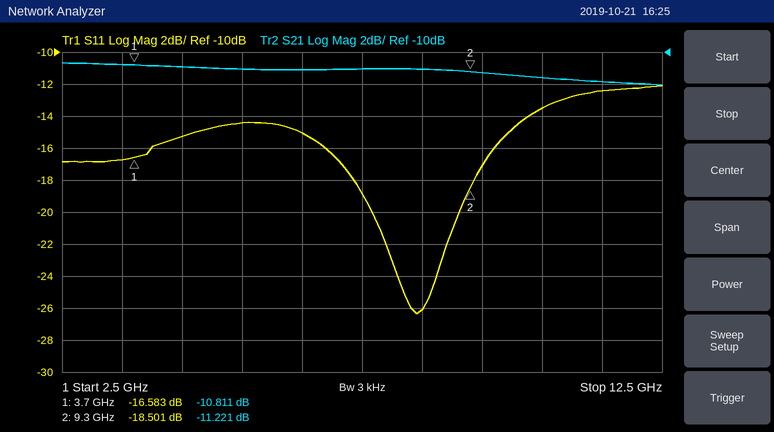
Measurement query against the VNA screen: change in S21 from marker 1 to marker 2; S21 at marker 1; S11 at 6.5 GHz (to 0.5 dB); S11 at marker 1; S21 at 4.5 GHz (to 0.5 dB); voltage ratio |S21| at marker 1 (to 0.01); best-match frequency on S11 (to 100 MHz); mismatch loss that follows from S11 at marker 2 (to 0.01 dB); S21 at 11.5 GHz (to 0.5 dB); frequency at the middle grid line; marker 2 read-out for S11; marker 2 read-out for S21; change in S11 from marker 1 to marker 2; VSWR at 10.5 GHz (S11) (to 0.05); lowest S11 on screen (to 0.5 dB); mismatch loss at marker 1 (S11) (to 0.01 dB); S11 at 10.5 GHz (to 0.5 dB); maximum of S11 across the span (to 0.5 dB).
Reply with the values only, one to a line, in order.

-0.410 dB
-10.811 dB
-15.0 dB
-16.583 dB
-11.0 dB
0.29
8.4 GHz
0.06 dB
-12.0 dB
7.5 GHz
-18.501 dB
-11.221 dB
-1.918 dB
1.55
-26.5 dB
0.10 dB
-13.5 dB
-12.0 dB
